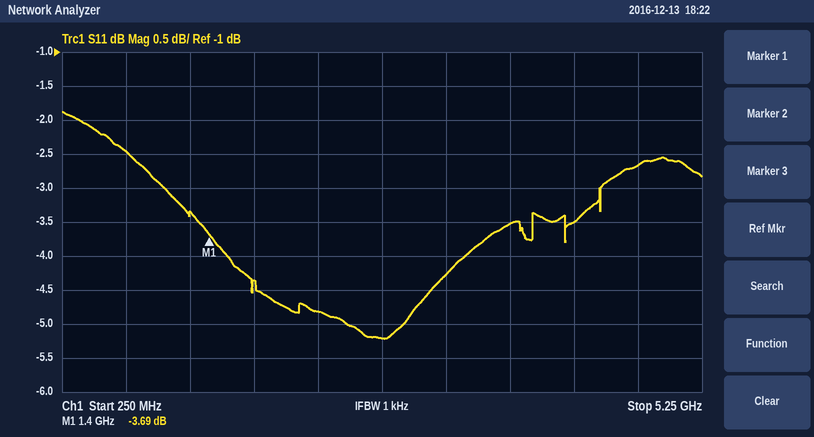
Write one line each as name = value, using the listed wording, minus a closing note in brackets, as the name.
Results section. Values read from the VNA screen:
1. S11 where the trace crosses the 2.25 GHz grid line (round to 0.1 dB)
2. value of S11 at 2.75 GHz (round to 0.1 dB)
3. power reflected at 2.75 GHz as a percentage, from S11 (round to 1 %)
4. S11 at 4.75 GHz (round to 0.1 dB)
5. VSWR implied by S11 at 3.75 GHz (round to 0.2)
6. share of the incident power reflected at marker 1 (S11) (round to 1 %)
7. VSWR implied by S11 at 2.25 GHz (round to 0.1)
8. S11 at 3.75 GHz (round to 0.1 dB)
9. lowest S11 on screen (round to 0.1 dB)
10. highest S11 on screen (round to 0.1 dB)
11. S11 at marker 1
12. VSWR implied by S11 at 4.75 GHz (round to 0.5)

S11 where the trace crosses the 2.25 GHz grid line = -4.8 dB
value of S11 at 2.75 GHz = -5.2 dB
power reflected at 2.75 GHz as a percentage, from S11 = 30 %
S11 at 4.75 GHz = -2.7 dB
VSWR implied by S11 at 3.75 GHz = 5.0
share of the incident power reflected at marker 1 (S11) = 43 %
VSWR implied by S11 at 2.25 GHz = 3.7
S11 at 3.75 GHz = -3.5 dB
lowest S11 on screen = -5.2 dB
highest S11 on screen = -1.9 dB
S11 at marker 1 = -3.69 dB
VSWR implied by S11 at 4.75 GHz = 6.5
